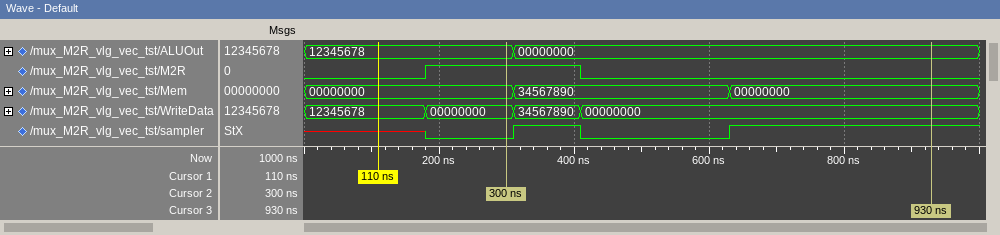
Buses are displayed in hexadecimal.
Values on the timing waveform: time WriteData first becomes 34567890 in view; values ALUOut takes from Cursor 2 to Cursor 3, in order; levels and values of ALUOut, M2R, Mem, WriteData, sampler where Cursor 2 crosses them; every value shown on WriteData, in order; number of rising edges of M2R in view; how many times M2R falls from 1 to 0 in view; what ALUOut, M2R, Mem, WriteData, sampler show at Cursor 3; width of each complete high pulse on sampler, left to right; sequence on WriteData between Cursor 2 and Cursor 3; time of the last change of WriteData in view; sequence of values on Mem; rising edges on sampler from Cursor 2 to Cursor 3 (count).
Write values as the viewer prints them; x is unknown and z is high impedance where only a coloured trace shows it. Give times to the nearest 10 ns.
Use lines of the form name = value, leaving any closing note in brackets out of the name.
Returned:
time WriteData first becomes 34567890 in view = 310 ns
values ALUOut takes from Cursor 2 to Cursor 3, in order = 12345678, 00000000
levels and values of ALUOut, M2R, Mem, WriteData, sampler where Cursor 2 crosses them = ALUOut=12345678, M2R=1, Mem=00000000, WriteData=00000000, sampler=0
every value shown on WriteData, in order = 12345678, 00000000, 34567890, 00000000
number of rising edges of M2R in view = 1
how many times M2R falls from 1 to 0 in view = 1
what ALUOut, M2R, Mem, WriteData, sampler show at Cursor 3 = ALUOut=00000000, M2R=0, Mem=00000000, WriteData=00000000, sampler=1
width of each complete high pulse on sampler, left to right = 100 ns
sequence on WriteData between Cursor 2 and Cursor 3 = 00000000, 34567890, 00000000
time of the last change of WriteData in view = 410 ns
sequence of values on Mem = 00000000, 34567890, 00000000
rising edges on sampler from Cursor 2 to Cursor 3 = 2
